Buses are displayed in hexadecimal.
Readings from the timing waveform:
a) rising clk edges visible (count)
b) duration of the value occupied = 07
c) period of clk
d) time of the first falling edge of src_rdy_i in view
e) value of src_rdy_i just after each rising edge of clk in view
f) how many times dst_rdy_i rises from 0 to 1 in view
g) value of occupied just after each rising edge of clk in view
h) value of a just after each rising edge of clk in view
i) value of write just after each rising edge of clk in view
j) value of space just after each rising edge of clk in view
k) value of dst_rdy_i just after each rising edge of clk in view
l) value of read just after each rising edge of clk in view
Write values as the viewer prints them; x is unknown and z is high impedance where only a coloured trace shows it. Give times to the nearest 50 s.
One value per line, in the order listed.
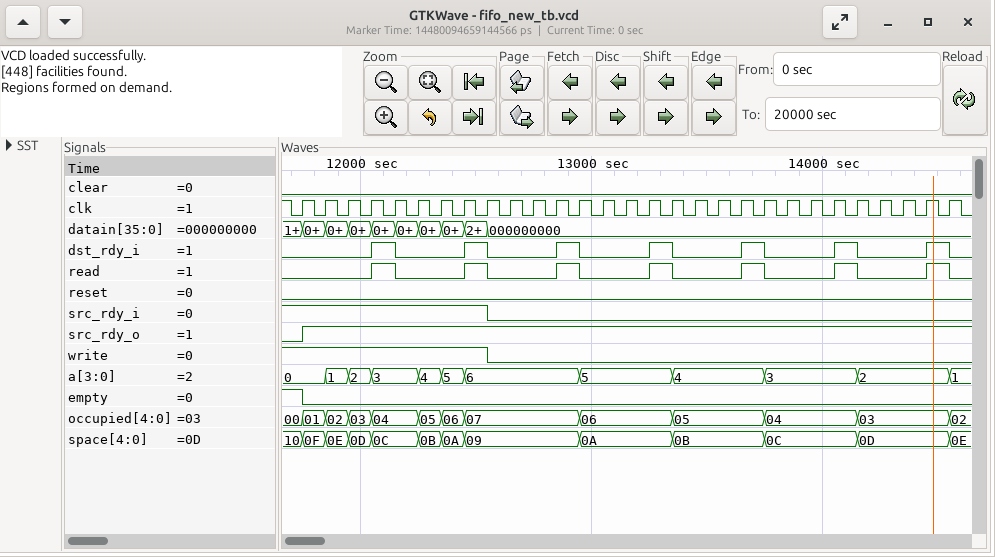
29
500 s
100 s
12550 s
1 1 1 1 1 1 1 1 0 0 0 0 0 0 0 0 0 0 0 0 0 0 0 0 0 0 0 0 0
7
01, 02, 03, 04, 04, 05, 06, 07, 07, 07, 07, 07, 06, 06, 06, 06, 05, 05, 05, 05, 04, 04, 04, 04, 03, 03, 03, 03, 02
0, 1, 2, 3, 3, 4, 5, 6, 6, 6, 6, 6, 5, 5, 5, 5, 4, 4, 4, 4, 3, 3, 3, 3, 2, 2, 2, 2, 1
1 1 1 1 1 1 1 1 0 0 0 0 0 0 0 0 0 0 0 0 0 0 0 0 0 0 0 0 0
0F, 0E, 0D, 0C, 0C, 0B, 0A, 09, 09, 09, 09, 09, 0A, 0A, 0A, 0A, 0B, 0B, 0B, 0B, 0C, 0C, 0C, 0C, 0D, 0D, 0D, 0D, 0E
0 0 0 1 0 0 0 1 0 0 0 1 0 0 0 1 0 0 0 1 0 0 0 1 0 0 0 1 0
0 0 0 1 0 0 0 1 0 0 0 1 0 0 0 1 0 0 0 1 0 0 0 1 0 0 0 1 0
